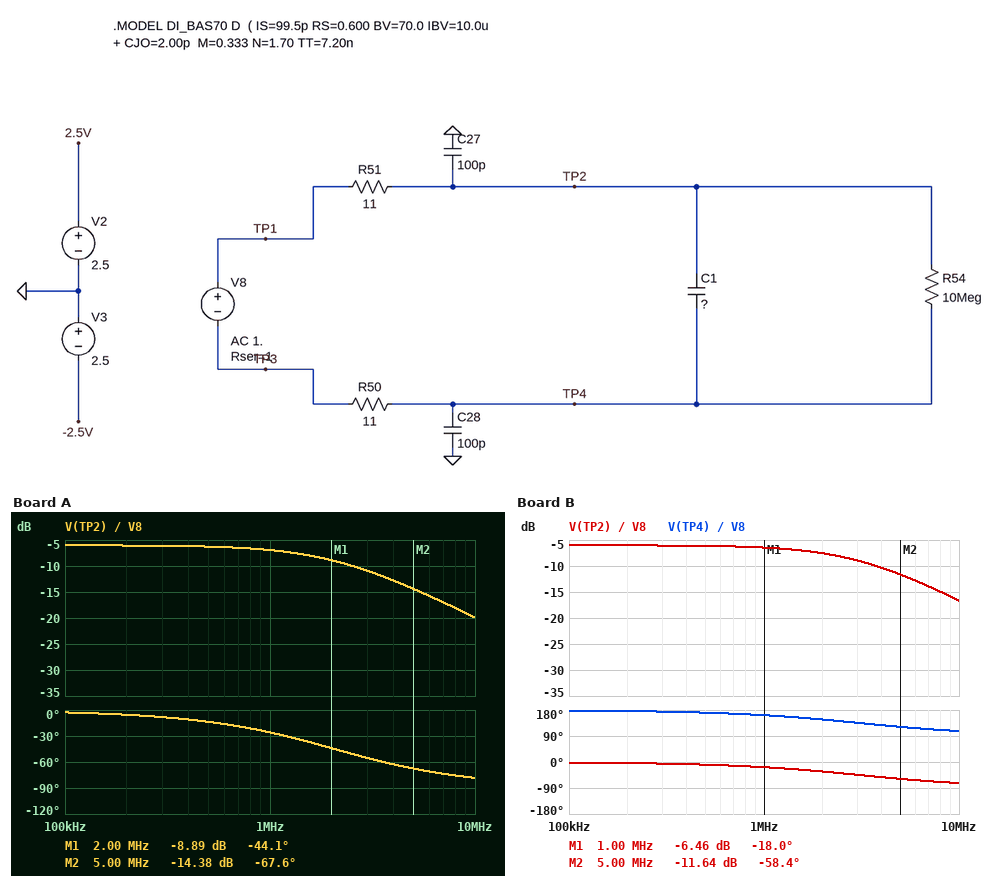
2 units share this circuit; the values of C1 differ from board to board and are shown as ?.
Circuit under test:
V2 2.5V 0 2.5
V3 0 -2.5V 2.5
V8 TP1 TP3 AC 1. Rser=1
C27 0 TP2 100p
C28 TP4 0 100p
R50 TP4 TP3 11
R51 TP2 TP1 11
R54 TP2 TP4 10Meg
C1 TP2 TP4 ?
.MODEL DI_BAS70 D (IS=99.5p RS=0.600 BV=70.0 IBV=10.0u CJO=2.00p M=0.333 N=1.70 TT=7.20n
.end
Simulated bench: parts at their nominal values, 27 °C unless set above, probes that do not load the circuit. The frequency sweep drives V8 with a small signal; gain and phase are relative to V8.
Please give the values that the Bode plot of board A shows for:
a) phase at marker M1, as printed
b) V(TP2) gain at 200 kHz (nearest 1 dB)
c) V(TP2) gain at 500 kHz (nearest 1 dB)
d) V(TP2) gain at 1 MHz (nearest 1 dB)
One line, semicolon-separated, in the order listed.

-44.1 deg; -6 dB; -6 dB; -7 dB
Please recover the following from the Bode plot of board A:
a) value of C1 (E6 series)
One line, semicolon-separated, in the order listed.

3.3 nF
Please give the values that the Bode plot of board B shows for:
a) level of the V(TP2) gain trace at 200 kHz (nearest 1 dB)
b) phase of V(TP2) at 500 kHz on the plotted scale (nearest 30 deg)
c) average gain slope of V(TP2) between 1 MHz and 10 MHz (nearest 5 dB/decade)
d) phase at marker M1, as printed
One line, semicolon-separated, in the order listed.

-6 dB; 0 deg; -10 dB/decade; -18.0 deg
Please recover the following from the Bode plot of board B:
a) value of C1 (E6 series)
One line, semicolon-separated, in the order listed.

2.2 nF
